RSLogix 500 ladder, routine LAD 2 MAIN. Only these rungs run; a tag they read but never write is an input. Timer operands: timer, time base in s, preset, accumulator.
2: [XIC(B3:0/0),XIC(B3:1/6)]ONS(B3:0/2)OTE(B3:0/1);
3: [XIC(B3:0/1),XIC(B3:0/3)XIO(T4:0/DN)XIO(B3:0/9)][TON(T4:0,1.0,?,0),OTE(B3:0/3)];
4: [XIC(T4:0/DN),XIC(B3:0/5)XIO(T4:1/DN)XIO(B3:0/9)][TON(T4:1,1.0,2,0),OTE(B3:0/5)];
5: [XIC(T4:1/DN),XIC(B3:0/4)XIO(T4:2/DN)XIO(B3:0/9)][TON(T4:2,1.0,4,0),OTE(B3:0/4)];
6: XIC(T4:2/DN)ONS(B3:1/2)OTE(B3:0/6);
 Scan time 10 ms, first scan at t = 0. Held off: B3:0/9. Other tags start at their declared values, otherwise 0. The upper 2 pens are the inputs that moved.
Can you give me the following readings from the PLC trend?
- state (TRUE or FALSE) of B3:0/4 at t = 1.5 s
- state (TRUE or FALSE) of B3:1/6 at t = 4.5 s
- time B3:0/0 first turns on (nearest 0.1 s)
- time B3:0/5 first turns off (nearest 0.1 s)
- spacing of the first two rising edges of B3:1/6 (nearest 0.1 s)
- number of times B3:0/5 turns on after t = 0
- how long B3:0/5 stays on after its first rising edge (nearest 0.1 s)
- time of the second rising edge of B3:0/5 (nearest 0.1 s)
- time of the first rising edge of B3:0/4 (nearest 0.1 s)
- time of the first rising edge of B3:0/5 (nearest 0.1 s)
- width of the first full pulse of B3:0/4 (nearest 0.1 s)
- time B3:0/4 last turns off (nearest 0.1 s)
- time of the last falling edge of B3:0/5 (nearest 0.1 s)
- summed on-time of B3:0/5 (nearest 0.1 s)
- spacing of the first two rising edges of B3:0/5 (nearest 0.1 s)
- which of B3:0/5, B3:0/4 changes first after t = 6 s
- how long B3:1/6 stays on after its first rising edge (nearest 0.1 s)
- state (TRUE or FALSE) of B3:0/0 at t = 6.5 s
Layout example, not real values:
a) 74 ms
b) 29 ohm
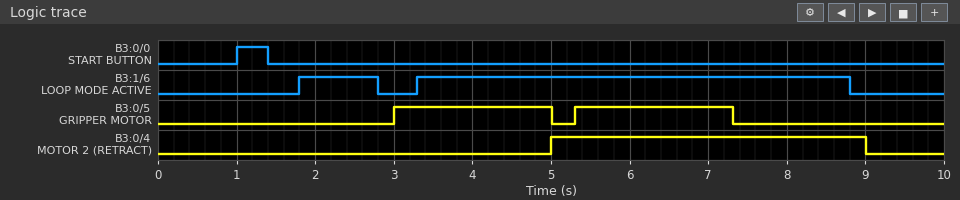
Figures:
a) FALSE
b) TRUE
c) 1.0 s
d) 5.0 s
e) 1.5 s
f) 2
g) 2.0 s
h) 5.3 s
i) 5.0 s
j) 3.0 s
k) 4.0 s
l) 9.0 s
m) 7.3 s
n) 4.0 s
o) 2.3 s
p) B3:0/5
q) 1.0 s
r) FALSE
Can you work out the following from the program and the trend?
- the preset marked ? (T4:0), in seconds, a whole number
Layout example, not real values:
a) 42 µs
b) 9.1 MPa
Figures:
a) 2 s
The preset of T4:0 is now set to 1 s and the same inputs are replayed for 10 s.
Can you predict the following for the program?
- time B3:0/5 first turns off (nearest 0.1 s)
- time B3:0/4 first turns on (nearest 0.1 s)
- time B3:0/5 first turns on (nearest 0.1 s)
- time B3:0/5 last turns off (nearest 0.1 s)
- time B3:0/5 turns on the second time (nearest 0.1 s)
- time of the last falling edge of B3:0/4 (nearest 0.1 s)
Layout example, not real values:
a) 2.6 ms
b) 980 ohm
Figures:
a) 4.0 s
b) 4.0 s
c) 2.0 s
d) 6.3 s
e) 4.3 s
f) 8.0 s
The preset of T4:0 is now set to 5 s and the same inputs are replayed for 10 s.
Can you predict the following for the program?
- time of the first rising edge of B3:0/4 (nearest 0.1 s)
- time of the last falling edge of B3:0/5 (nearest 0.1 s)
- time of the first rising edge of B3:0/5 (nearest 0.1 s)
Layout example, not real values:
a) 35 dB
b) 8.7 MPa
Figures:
a) 8.0 s
b) 8.0 s
c) 6.0 s
